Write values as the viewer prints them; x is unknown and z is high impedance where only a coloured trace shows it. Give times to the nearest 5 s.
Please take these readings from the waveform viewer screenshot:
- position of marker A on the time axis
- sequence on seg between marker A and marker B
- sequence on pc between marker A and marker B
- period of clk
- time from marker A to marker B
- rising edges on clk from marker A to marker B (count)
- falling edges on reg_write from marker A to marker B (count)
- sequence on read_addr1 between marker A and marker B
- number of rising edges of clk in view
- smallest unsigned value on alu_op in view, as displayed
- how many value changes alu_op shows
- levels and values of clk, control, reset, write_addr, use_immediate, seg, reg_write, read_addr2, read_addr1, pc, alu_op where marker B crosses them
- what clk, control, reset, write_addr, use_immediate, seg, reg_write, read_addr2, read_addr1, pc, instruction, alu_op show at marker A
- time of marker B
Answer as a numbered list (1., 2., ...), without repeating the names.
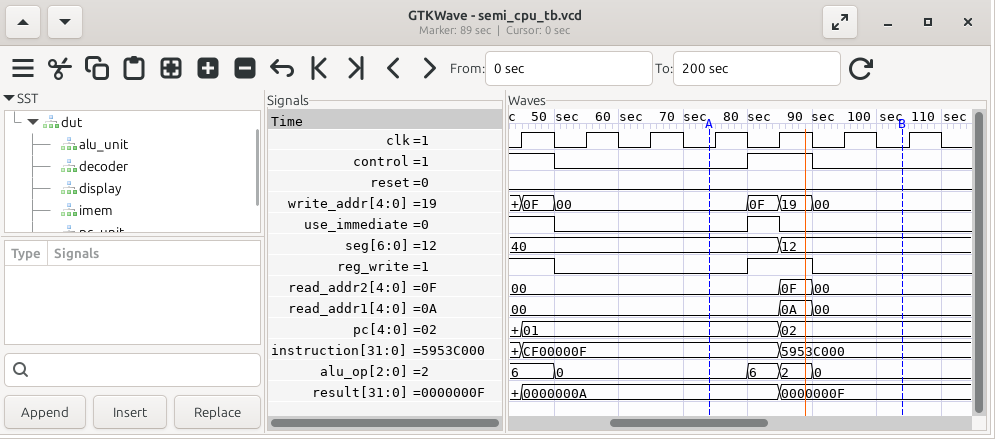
1. 75 s
2. 40, 12
3. 01, 02
4. 10 s
5. 30 s
6. 3
7. 1
8. 00, 0A, 00
9. 7
10. 0
11. 4
12. clk=0, control=0, reset=0, write_addr=00, use_immediate=0, seg=12, reg_write=0, read_addr2=00, read_addr1=00, pc=02, alu_op=0
13. clk=0, control=0, reset=0, write_addr=00, use_immediate=0, seg=40, reg_write=0, read_addr2=00, read_addr1=00, pc=01, instruction=CF00000F, alu_op=0
14. 105 s
